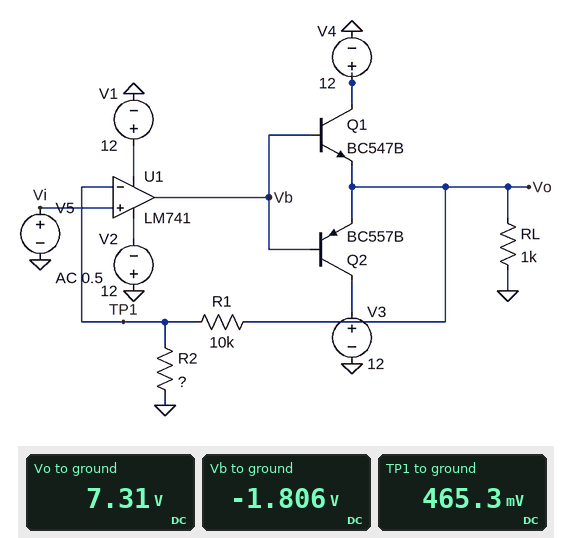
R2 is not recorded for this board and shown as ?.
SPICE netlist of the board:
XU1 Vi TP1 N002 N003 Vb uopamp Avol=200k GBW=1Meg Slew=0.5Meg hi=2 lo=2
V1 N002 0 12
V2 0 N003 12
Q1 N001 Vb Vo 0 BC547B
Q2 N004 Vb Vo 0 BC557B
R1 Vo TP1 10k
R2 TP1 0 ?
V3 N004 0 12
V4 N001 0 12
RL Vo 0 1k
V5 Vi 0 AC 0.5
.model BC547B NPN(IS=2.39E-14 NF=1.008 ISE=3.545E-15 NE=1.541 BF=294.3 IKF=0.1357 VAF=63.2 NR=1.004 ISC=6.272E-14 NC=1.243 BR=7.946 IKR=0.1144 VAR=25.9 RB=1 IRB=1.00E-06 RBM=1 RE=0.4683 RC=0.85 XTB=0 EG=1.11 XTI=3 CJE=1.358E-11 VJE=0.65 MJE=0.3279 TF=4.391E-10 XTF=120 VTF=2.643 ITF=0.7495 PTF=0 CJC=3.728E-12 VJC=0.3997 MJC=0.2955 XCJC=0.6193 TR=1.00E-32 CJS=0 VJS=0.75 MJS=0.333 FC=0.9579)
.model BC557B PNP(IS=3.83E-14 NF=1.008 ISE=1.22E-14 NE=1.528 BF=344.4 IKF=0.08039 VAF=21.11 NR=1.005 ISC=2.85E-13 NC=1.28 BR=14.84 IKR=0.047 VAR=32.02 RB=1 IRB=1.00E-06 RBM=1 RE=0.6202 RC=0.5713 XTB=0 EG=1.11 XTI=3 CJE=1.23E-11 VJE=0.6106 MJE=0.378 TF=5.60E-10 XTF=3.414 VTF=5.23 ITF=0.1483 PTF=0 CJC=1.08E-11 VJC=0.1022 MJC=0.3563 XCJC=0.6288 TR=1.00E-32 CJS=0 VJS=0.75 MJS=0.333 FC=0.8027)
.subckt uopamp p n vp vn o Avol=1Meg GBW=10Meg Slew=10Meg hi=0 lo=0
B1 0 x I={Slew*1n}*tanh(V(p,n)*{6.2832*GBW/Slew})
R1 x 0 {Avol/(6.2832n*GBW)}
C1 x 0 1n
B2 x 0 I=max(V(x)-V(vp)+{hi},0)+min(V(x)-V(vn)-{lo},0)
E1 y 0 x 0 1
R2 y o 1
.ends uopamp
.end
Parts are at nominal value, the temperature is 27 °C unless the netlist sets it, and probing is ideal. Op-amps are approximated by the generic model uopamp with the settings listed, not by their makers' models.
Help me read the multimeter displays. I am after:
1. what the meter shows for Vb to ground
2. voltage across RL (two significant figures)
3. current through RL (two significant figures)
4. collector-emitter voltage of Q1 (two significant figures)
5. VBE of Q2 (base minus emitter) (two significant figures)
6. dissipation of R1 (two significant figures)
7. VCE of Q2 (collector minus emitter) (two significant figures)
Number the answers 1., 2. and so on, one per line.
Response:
1. -1.806 V
2. 7.3 V
3. 7.3 mA
4. 4.7 V
5. -9.1 V
6. 4.7 mW
7. 4.7 V
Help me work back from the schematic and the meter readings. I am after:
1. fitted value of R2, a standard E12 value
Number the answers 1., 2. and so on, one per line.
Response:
1. 680 Ω
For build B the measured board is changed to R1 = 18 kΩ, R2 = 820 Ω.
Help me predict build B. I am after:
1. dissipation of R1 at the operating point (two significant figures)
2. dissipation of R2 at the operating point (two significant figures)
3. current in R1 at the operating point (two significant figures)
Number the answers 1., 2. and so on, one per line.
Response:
1. 2.7 mW
2. 120 µW
3. 390 µA
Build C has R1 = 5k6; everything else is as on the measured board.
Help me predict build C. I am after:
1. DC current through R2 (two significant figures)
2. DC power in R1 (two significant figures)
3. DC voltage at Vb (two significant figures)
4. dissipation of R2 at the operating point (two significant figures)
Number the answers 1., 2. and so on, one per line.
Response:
1. 1.2 mA
2. 7.6 mW
3. -1.8 V
4. 920 µW
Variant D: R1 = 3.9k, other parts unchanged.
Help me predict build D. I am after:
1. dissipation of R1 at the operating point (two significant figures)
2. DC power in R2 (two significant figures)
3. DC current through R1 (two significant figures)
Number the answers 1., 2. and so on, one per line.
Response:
1. 9.9 mW
2. 1.7 mW
3. 1.6 mA
